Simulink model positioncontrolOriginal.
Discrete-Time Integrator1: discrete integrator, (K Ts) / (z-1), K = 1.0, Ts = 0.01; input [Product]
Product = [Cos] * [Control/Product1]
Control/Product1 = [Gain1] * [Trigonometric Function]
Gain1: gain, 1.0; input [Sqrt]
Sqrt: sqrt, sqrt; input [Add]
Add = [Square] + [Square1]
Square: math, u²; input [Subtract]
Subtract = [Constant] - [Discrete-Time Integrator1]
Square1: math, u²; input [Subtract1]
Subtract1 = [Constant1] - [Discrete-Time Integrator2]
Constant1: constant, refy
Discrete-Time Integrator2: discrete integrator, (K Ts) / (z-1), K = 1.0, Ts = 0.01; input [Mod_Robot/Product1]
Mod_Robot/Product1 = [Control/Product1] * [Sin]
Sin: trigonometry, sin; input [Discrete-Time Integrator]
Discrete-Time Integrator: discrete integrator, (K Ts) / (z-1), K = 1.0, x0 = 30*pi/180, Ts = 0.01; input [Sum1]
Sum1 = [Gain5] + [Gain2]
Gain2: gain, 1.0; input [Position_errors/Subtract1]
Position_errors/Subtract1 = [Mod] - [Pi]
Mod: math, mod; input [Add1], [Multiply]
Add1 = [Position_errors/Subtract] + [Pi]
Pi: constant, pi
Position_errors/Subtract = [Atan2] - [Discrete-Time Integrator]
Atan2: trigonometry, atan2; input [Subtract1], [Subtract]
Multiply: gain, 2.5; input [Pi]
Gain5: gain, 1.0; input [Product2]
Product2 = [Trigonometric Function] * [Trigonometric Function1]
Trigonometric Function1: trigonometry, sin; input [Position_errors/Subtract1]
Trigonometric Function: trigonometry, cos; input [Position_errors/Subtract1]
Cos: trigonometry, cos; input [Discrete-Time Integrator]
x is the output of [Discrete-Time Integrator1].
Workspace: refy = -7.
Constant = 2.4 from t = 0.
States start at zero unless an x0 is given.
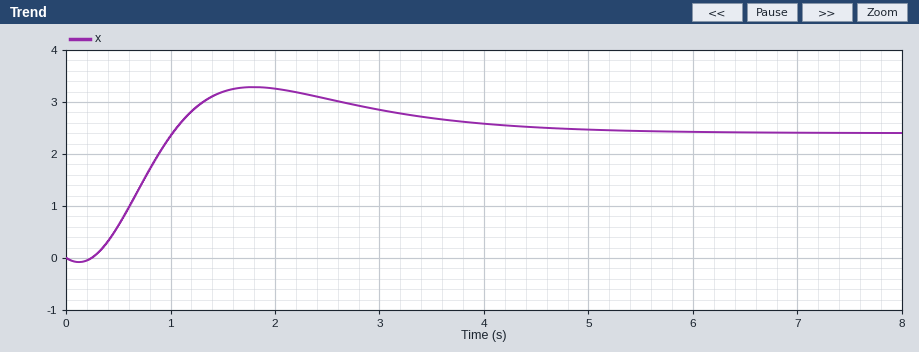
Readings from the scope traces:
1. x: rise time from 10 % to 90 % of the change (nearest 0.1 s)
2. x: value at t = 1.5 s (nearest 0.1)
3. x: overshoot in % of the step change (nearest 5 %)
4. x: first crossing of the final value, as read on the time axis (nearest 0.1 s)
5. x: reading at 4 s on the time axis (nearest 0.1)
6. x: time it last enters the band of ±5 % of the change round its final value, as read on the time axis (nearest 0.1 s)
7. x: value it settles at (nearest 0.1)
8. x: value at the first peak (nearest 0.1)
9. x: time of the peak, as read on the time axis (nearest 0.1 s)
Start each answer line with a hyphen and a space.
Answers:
- 0.6 s
- 3.2
- 35 %
- 1.0 s
- 2.6
- 4.4 s
- 2.4
- 3.3
- 1.8 s
